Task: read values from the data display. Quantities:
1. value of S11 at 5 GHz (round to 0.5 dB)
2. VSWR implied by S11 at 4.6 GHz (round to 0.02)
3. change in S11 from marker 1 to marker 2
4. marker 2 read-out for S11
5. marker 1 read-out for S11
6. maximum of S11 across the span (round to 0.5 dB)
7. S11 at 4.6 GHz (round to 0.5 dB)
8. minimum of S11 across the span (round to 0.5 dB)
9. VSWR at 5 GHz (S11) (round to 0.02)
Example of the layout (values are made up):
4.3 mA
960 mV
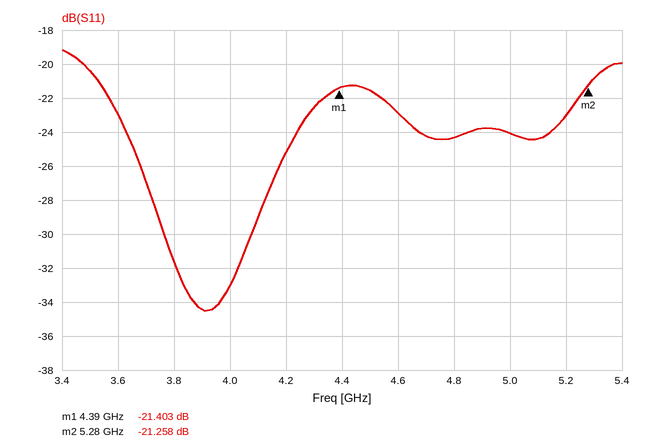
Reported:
-24.0 dB
1.16
0.145 dB
-21.258 dB
-21.403 dB
-19.0 dB
-23.0 dB
-34.5 dB
1.14
